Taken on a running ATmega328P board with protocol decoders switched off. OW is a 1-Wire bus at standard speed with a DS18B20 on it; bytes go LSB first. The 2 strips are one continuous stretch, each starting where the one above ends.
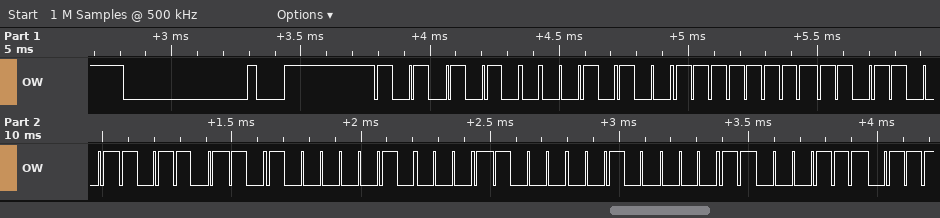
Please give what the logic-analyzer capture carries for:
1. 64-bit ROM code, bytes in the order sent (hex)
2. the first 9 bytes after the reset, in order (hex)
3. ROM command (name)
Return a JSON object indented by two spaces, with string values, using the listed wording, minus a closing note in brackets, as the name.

{
  "64-bit ROM code, bytes in the order sent": "28 FF 9B 6D 41 18 04 E3",
  "the first 9 bytes after the reset, in order": "55 28 FF 9B 6D 41 18 04 E3",
  "ROM command": "Match ROM"
}
